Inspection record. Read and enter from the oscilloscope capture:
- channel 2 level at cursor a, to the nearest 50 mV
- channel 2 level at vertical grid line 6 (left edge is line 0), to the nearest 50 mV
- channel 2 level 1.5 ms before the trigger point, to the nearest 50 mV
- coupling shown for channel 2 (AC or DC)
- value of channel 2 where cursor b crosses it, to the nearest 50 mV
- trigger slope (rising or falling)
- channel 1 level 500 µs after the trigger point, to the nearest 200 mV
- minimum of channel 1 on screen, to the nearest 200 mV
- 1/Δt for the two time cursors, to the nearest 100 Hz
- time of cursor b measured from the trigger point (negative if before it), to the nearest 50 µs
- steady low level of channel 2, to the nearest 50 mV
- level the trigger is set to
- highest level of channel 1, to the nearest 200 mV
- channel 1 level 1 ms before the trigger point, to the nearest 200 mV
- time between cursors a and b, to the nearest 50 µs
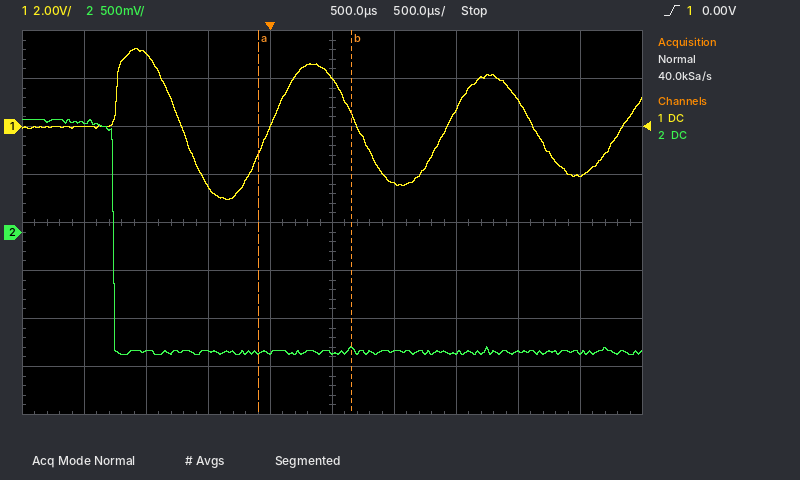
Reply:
-1.25 V
-1.25 V
1.15 V
DC
-1.20 V
rising
2.0 V
-3.0 V
1.3 kHz
+650 µs
-1.25 V
0.00 V
3.2 V
3.0 V
750 µs
